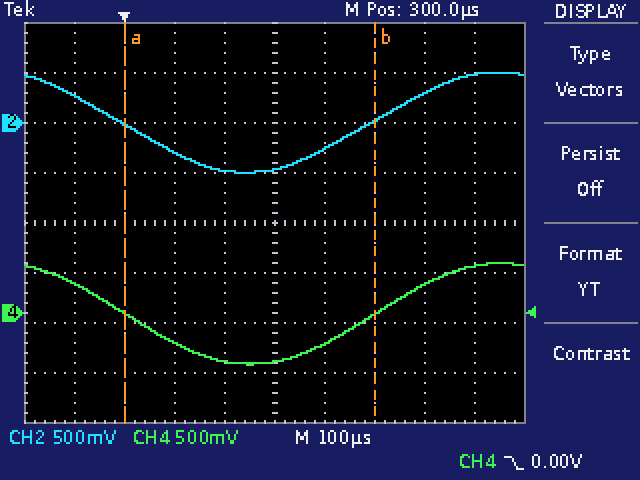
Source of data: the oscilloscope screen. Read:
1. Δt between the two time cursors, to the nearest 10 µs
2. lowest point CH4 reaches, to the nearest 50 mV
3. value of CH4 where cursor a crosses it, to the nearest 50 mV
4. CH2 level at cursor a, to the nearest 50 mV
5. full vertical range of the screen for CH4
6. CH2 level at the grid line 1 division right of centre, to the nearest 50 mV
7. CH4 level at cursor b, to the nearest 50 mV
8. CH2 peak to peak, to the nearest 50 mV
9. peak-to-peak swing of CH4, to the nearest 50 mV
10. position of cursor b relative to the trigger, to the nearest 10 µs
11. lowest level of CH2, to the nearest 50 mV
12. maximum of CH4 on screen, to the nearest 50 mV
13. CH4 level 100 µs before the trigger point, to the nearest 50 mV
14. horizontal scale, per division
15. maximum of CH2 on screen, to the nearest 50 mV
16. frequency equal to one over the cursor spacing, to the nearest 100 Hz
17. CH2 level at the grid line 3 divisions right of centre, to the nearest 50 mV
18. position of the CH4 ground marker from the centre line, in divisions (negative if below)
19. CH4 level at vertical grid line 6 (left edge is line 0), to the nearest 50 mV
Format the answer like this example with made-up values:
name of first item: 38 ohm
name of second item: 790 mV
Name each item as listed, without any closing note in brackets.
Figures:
Δt between the two time cursors, to the nearest 10 µs: 500 µs
lowest point CH4 reaches, to the nearest 50 mV: -500 mV
value of CH4 where cursor a crosses it, to the nearest 50 mV: 0 mV
CH2 level at cursor a, to the nearest 50 mV: 0 mV
full vertical range of the screen for CH4: 4 V
CH2 level at the grid line 1 division right of centre, to the nearest 50 mV: -250 mV
CH4 level at cursor b, to the nearest 50 mV: 0 mV
CH2 peak to peak, to the nearest 50 mV: 1.00 V
peak-to-peak swing of CH4, to the nearest 50 mV: 1.00 V
position of cursor b relative to the trigger, to the nearest 10 µs: +500 µs
lowest level of CH2, to the nearest 50 mV: -500 mV
maximum of CH4 on screen, to the nearest 50 mV: 500 mV
CH4 level 100 µs before the trigger point, to the nearest 50 mV: 300 mV
horizontal scale, per division: 100 µs
maximum of CH2 on screen, to the nearest 50 mV: 500 mV
frequency equal to one over the cursor spacing, to the nearest 100 Hz: 2.0 kHz
CH2 level at the grid line 3 divisions right of centre, to the nearest 50 mV: 300 mV
position of the CH4 ground marker from the centre line, in divisions: -1.8 div
CH4 level at vertical grid line 6 (left edge is line 0), to the nearest 50 mV: -300 mV
